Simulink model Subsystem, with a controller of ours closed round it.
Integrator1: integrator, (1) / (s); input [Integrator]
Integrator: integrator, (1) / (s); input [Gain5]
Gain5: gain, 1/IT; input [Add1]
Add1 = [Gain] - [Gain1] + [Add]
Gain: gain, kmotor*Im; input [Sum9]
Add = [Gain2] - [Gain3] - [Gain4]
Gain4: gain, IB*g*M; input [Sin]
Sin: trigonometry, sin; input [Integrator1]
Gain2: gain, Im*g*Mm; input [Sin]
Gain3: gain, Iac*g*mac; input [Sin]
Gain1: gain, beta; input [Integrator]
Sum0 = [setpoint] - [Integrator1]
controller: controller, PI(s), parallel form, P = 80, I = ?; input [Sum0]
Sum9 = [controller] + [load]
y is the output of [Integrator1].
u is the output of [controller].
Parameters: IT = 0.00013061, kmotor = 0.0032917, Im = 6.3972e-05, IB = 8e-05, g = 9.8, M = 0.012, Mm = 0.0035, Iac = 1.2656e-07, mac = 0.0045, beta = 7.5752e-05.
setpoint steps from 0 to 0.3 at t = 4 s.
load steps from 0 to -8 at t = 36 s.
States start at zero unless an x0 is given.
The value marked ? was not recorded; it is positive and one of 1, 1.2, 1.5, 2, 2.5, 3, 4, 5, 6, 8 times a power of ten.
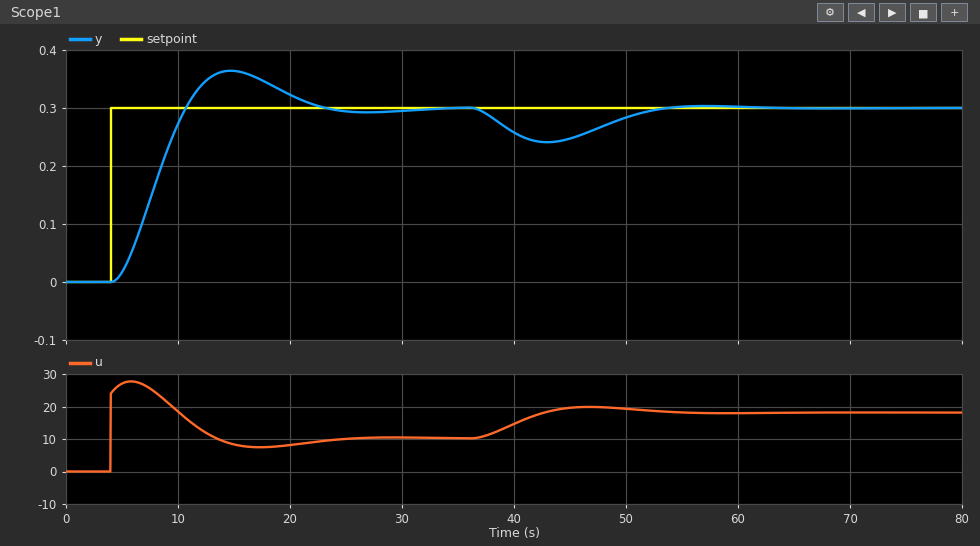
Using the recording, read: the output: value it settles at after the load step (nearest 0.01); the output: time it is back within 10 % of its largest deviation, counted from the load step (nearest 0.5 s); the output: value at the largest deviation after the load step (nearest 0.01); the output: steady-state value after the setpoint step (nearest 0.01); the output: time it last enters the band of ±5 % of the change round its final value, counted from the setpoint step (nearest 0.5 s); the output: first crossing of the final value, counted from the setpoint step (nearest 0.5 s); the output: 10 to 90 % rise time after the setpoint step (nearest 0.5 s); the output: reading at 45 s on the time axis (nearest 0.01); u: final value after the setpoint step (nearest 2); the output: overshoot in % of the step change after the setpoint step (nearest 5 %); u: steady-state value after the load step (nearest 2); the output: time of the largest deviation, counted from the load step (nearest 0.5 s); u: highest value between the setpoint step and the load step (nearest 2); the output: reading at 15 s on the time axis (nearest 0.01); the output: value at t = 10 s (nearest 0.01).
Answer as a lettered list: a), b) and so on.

a) 0.30
b) 16.0 s
c) 0.24
d) 0.30
e) 17.0 s
f) 6.5 s
g) 4.5 s
h) 0.25
i) 10
j) 20 %
k) 18
l) 7.0 s
m) 28
n) 0.36
o) 0.27
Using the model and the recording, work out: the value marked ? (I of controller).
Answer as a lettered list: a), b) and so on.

a) 15
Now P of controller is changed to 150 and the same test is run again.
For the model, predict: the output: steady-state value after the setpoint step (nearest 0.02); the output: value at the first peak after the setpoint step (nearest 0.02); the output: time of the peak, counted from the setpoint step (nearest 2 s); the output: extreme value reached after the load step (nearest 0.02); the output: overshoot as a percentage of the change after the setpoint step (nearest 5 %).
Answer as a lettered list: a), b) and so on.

a) 0.30
b) 0.34
c) 8 s
d) 0.26
e) 15 %
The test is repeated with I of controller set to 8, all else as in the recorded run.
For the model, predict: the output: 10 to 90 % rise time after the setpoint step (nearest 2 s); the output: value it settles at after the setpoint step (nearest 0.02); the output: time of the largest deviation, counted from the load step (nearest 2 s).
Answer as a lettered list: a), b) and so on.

a) 6 s
b) 0.30
c) 8 s
